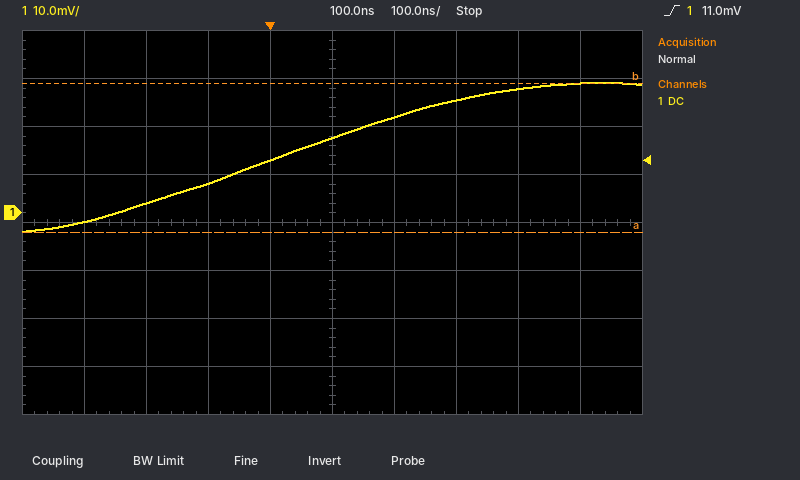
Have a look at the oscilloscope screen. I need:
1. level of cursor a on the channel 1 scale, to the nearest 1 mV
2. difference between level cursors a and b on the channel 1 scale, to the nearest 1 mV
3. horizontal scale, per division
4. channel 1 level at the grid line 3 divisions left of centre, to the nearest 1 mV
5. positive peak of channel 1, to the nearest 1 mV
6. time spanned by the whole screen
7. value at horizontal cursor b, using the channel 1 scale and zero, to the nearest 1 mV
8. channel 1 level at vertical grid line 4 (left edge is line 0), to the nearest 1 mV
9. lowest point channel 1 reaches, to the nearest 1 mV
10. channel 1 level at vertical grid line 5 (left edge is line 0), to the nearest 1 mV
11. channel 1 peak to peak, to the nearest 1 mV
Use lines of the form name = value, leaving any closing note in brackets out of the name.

level of cursor a on the channel 1 scale, to the nearest 1 mV = -4 mV
difference between level cursors a and b on the channel 1 scale, to the nearest 1 mV = 31 mV
horizontal scale, per division = 100 ns
channel 1 level at the grid line 3 divisions left of centre, to the nearest 1 mV = 2 mV
positive peak of channel 1, to the nearest 1 mV = 27 mV
time spanned by the whole screen = 1 µs
value at horizontal cursor b, using the channel 1 scale and zero, to the nearest 1 mV = 27 mV
channel 1 level at vertical grid line 4 (left edge is line 0), to the nearest 1 mV = 11 mV
lowest point channel 1 reaches, to the nearest 1 mV = -4 mV
channel 1 level at vertical grid line 5 (left edge is line 0), to the nearest 1 mV = 16 mV
channel 1 peak to peak, to the nearest 1 mV = 31 mV
